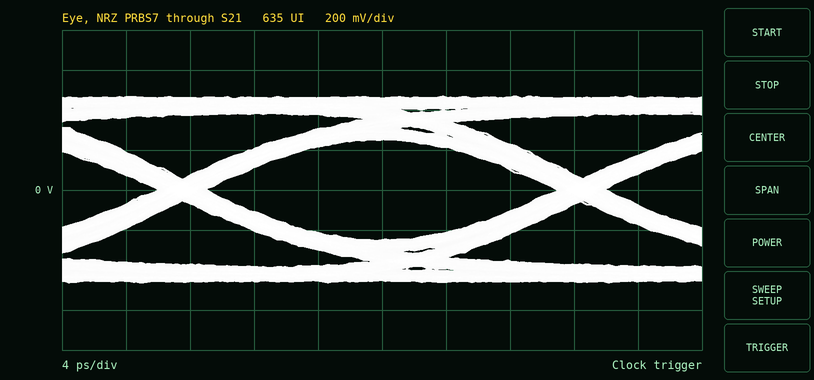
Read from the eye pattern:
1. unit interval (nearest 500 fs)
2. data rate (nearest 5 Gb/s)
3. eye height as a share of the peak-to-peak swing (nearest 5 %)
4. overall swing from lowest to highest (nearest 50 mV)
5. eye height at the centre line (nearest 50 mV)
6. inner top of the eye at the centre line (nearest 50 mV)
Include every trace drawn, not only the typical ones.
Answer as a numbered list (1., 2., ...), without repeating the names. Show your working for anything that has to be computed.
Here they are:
1. 25.0 ps
2. 40 Gb/s
3. 500 mV / 950 mV ≈ 52.6 %, so 55 % to the nearest 5 %
4. 950 mV
5. 500 mV
6. 250 mV
